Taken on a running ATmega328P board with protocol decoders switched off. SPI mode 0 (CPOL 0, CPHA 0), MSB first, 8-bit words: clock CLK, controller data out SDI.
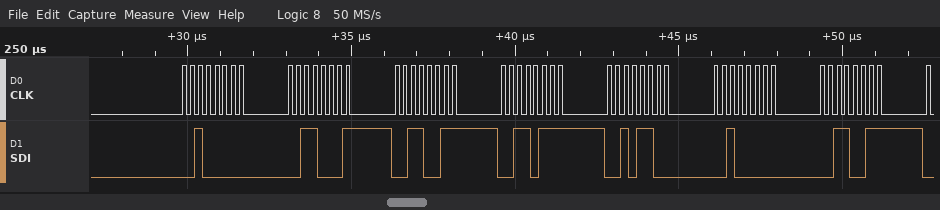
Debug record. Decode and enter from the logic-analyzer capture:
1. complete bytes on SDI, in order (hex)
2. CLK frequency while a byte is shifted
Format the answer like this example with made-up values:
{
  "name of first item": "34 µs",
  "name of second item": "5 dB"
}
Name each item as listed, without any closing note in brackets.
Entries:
{
  "complete bytes on SDI, in order": "20 31 33 37 2C 20 33",
  "CLK frequency while a byte is shifted": "4 MHz"
}
